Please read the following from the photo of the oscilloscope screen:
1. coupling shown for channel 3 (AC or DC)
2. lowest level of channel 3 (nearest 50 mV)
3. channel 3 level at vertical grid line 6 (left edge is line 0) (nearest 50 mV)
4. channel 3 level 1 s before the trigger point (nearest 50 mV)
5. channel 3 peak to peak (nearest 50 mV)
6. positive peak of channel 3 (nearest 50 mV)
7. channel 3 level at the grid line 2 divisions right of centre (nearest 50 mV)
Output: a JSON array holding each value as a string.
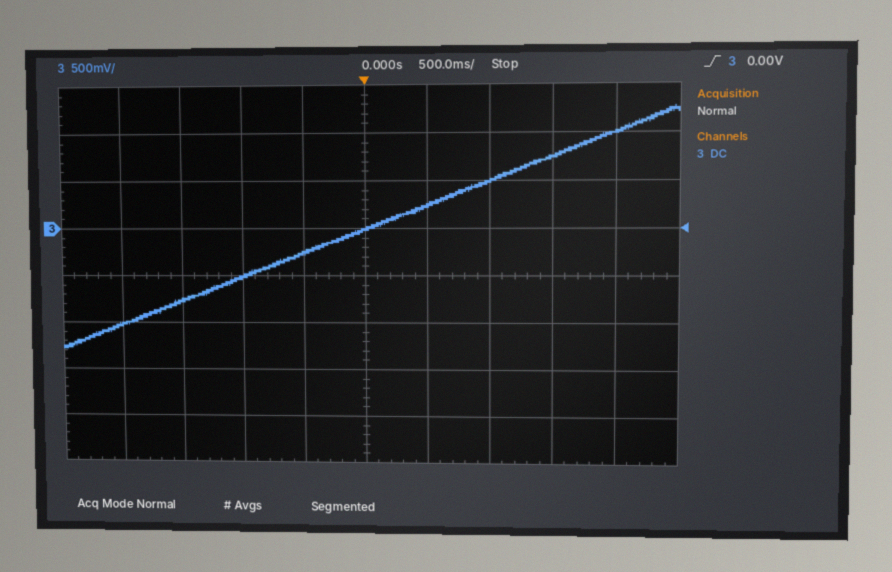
["DC", "-1.30 V", "250 mV", "-500 mV", "2.55 V", "1.25 V", "500 mV"]
